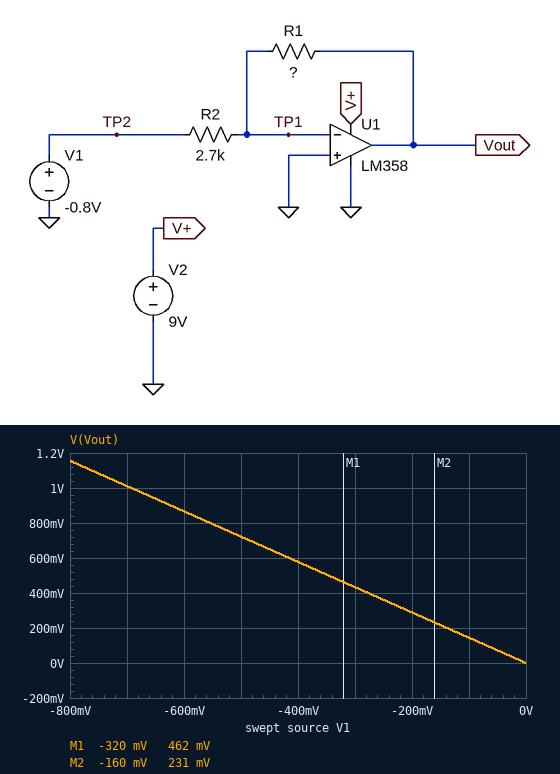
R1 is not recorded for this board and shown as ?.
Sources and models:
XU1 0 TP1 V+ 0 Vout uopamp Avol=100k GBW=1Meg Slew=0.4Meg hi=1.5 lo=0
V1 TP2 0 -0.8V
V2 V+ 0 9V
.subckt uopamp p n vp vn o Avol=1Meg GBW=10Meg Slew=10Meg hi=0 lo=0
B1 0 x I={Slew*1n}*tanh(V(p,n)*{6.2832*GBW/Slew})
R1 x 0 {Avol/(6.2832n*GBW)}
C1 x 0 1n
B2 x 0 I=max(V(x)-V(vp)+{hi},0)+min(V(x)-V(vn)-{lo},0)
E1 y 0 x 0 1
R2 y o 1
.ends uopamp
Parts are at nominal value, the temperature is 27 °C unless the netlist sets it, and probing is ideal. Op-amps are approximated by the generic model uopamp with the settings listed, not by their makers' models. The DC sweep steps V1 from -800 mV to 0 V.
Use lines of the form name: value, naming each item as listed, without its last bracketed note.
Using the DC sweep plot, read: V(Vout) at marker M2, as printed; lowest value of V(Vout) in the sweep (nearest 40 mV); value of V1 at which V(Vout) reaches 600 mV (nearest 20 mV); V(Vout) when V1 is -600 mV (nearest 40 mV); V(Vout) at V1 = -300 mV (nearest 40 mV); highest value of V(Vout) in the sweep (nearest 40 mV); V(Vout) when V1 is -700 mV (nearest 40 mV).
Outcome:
V(Vout) at marker M2, as printed: 231 mV
lowest value of V(Vout) in the sweep: 0 V
value of V1 at which V(Vout) reaches 600 mV: -420 mV
V(Vout) when V1 is -600 mV: 880 mV
V(Vout) at V1 = -300 mV: 440 mV
highest value of V(Vout) in the sweep: 1.16 V
V(Vout) when V1 is -700 mV: 1.00 V
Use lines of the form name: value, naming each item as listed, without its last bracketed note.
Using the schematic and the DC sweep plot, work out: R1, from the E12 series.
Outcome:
R1, from the E12 series: 3.9 kΩ
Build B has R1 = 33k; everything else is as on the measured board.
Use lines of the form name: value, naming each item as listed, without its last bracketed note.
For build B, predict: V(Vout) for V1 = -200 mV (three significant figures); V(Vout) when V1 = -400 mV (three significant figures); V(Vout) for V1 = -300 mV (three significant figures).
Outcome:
V(Vout) for V1 = -200 mV: 2.44 V
V(Vout) when V1 = -400 mV: 4.89 V
V(Vout) for V1 = -300 mV: 3.67 V
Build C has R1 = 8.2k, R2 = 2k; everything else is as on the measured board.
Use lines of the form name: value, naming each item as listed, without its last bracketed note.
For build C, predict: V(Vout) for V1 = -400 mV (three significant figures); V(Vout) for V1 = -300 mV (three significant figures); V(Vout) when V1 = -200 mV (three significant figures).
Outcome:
V(Vout) for V1 = -400 mV: 1.64 V
V(Vout) for V1 = -300 mV: 1.23 V
V(Vout) when V1 = -200 mV: 820 mV
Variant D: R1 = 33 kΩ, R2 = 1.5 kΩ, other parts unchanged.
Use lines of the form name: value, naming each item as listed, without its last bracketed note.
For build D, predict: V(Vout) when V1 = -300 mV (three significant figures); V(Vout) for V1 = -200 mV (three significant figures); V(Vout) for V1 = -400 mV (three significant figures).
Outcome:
V(Vout) when V1 = -300 mV: 6.60 V
V(Vout) for V1 = -200 mV: 4.40 V
V(Vout) for V1 = -400 mV: 7.50 V
